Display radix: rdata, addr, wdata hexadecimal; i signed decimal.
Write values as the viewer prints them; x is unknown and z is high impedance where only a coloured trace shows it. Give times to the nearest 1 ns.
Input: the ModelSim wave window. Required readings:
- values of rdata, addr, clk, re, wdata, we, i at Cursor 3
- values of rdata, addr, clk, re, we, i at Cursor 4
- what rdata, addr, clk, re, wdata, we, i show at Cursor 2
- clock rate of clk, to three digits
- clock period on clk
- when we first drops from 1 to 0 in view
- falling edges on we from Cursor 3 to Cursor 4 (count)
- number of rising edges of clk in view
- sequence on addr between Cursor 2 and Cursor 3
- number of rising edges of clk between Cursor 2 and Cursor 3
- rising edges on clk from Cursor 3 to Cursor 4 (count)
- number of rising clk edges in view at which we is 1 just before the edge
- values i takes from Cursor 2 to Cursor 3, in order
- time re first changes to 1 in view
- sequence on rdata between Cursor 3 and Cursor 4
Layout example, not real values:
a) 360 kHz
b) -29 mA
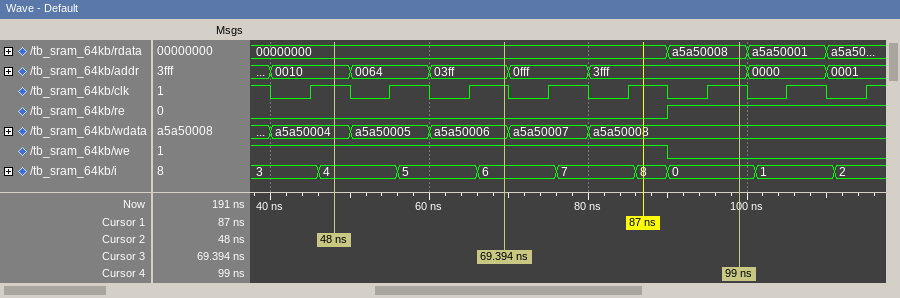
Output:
a) rdata=00000000, addr=03ff, clk=1, re=0, wdata=a5a50006, we=1, i=6
b) rdata=a5a50008, addr=3fff, clk=1, re=1, we=0, i=0
c) rdata=00000000, addr=0010, clk=1, re=0, wdata=a5a50004, we=1, i=4
d) 100 MHz
e) 10 ns
f) 90 ns
g) 1
h) 8
i) 0010, 0064, 03ff
j) 2
k) 3
l) 5
m) 4, 5, 6
n) 90 ns
o) 00000000, a5a50008
